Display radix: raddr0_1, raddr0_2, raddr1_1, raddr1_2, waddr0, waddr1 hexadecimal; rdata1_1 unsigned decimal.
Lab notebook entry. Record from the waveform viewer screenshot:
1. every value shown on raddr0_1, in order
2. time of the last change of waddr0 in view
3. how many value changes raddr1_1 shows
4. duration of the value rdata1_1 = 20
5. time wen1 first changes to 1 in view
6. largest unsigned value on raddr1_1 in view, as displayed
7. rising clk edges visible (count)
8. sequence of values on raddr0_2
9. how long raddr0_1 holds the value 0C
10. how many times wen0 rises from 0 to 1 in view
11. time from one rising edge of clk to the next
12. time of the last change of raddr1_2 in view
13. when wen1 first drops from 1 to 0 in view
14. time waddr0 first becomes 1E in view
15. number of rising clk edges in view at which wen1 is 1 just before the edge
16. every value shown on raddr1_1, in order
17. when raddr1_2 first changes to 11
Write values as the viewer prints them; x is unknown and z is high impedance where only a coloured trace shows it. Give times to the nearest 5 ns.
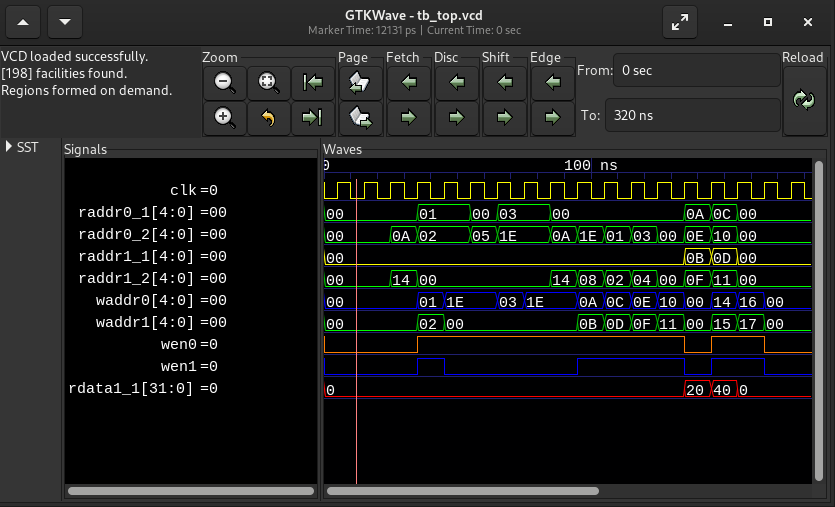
00, 01, 00, 03, 00, 0A, 0C, 00
165 ns
3
10 ns
35 ns
0D
18
00, 0A, 02, 05, 1E, 0A, 1E, 01, 03, 00, 0E, 10, 00
10 ns
2
10 ns
155 ns
45 ns
45 ns
7
00, 0B, 0D, 00
145 ns
